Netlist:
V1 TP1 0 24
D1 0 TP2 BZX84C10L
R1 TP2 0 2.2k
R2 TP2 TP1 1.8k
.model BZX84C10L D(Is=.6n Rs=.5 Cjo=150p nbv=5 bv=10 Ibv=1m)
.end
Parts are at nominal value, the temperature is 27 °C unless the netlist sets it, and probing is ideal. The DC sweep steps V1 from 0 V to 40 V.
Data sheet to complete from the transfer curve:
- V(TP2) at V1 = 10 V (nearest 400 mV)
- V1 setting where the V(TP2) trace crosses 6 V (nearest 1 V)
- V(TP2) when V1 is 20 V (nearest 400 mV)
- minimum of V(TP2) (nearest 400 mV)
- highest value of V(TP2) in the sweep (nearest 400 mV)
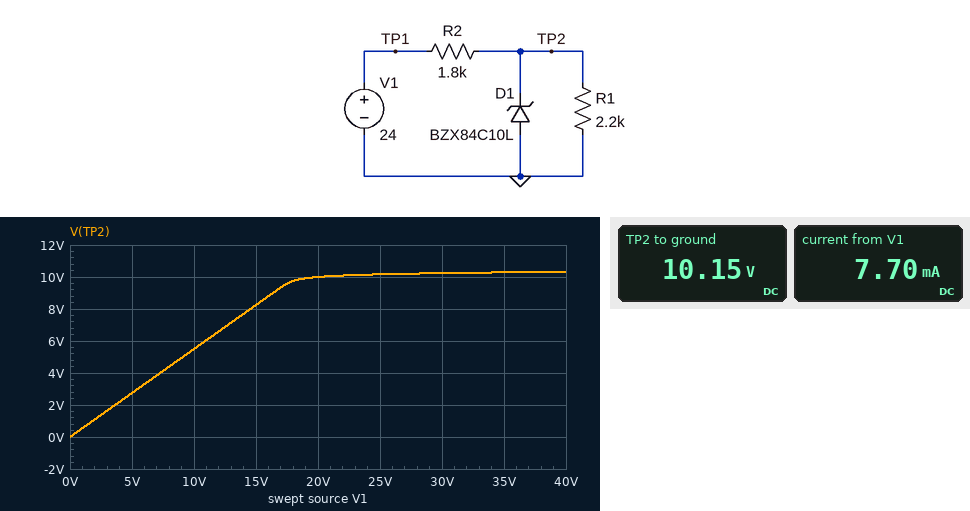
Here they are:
5.6 V
11 V
10.0 V
0 V
10.4 V
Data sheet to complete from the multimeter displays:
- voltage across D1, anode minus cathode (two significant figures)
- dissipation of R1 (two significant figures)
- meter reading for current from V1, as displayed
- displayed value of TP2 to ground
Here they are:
-10 V
47 mW
7.70 mA
10.15 V
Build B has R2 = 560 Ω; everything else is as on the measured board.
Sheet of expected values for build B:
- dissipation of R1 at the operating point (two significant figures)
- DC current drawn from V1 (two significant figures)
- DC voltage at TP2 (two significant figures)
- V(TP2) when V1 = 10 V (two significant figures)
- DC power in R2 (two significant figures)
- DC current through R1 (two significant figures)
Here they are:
49 mW
24 mA
10 V
8.0 V
330 mW
4.7 mA
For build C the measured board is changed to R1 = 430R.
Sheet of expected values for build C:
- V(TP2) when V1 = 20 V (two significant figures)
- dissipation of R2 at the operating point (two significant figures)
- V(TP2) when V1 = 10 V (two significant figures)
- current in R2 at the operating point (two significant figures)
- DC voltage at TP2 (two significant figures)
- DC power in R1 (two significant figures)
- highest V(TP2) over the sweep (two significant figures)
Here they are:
3.9 V
210 mW
1.9 V
11 mA
4.6 V
50 mW
7.7 V
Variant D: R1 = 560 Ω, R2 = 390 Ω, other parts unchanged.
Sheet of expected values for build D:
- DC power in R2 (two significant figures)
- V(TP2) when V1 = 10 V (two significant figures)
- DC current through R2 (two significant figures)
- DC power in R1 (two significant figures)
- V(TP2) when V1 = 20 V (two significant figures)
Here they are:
480 mW
5.9 V
35 mA
190 mW
10 V
